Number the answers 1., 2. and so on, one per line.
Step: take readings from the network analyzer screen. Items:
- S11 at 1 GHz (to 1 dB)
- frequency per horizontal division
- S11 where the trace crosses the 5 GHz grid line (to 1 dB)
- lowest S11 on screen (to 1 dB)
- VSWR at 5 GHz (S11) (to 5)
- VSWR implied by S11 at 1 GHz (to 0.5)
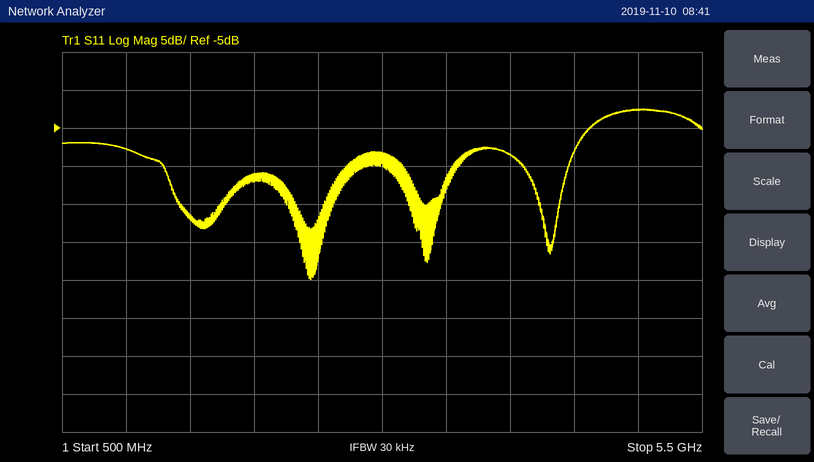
1. -8 dB
2. 500 MHz
3. -3 dB
4. -25 dB
5. 5
6. 2.5
